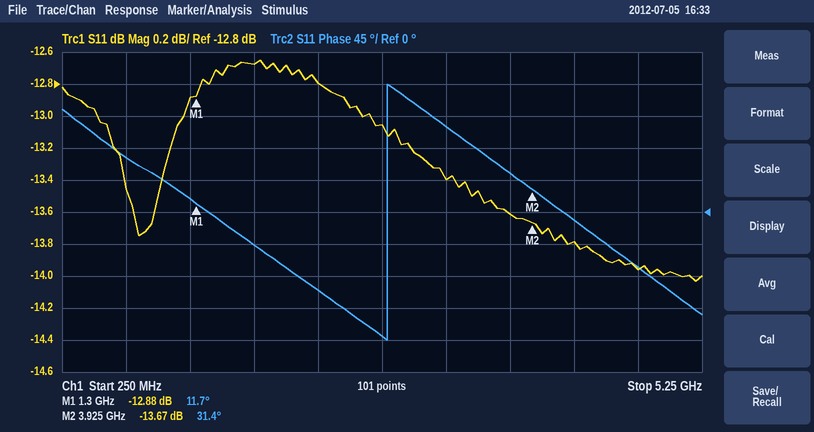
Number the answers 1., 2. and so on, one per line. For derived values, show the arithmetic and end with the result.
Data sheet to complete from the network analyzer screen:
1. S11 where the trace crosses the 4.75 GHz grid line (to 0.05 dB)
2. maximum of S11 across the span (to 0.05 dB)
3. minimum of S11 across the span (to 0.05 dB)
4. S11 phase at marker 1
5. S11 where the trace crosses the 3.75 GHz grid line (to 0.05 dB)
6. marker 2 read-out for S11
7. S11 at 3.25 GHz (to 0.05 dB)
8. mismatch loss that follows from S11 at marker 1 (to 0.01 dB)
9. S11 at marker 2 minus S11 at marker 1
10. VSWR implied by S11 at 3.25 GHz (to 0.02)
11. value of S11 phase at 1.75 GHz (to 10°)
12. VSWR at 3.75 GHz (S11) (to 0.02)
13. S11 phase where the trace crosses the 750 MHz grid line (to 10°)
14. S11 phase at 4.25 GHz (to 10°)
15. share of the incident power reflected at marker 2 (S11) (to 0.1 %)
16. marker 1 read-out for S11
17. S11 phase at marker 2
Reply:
1. -13.95 dB
2. -12.65 dB
3. -14.05 dB
4. 11.7°
5. -13.60 dB
6. -13.67 dB
7. -13.40 dB
8. −10 log10(1 − 10^(-12.88/10)) ≈ 0.23 dB
9. -13.67 − (-12.88) = -0.79 dB
10. |Γ| = 10^(-13.4/20) = 0.2138; VSWR = (1 + 0.2138)/(1 − 0.2138) ≈ 1.54
11. -50°
12. |Γ| = 10^(-13.6/20) = 0.2089; VSWR = (1 + 0.2089)/(1 − 0.2089) ≈ 1.53, so 1.52 to the nearest 0.02
13. 80°
14. -10°
15. 10^(-13.67/10) ≈ 4.3 %
16. -12.88 dB
17. 31.4°
